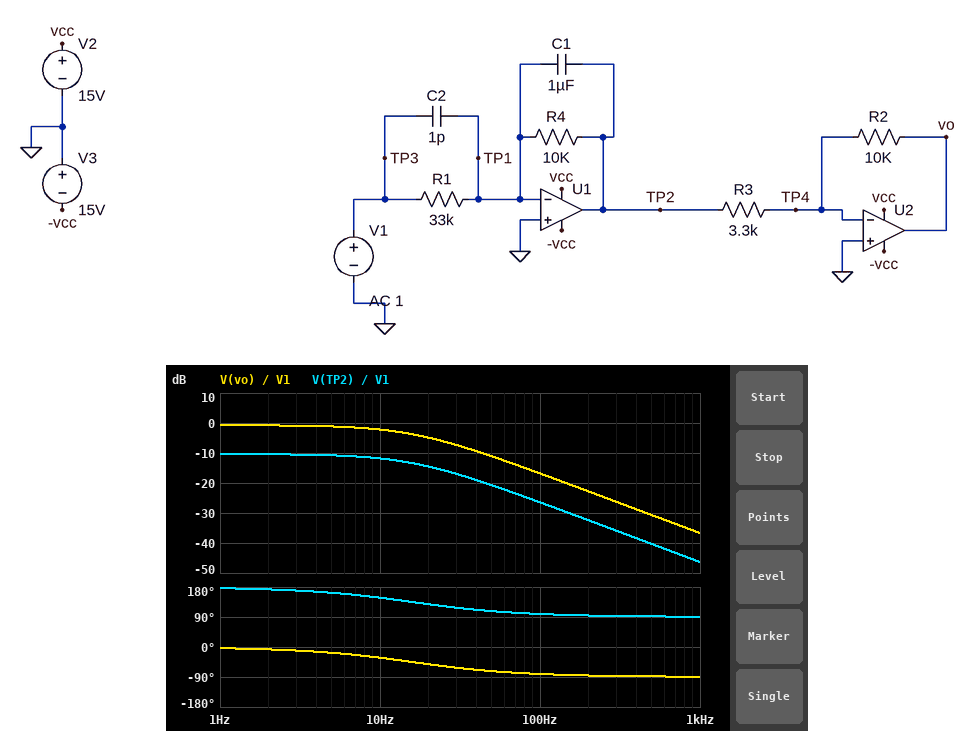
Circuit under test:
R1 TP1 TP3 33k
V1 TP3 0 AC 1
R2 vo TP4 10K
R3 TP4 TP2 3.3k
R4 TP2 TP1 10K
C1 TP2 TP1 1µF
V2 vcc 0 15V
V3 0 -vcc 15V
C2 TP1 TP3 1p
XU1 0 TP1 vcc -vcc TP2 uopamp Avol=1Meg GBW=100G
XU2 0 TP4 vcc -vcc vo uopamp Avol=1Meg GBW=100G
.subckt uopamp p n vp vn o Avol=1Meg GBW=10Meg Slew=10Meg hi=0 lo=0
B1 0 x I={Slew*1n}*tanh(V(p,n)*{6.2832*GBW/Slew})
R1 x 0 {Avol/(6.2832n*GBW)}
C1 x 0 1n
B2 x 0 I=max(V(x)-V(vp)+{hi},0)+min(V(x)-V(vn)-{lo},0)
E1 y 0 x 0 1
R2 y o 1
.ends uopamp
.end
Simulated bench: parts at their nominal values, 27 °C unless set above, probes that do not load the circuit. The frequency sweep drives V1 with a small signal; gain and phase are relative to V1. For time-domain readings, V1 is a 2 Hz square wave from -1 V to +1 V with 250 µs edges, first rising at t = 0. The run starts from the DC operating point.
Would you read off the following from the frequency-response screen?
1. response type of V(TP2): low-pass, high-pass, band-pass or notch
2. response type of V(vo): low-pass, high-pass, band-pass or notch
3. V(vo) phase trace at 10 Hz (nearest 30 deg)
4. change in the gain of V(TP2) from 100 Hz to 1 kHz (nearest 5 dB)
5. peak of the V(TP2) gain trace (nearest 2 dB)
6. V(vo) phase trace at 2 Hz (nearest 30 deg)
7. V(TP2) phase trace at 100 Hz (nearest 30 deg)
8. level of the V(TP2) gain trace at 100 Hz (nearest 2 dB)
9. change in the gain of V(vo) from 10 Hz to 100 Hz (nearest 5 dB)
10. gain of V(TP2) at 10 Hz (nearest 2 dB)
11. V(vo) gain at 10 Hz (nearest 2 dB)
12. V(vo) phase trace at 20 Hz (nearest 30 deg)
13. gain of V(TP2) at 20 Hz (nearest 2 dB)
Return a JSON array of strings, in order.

["low-pass", "low-pass", "-30 deg", "-20 dB", "-10 dB", "0 deg", "90 deg", "-26 dB", "-15 dB", "-12 dB", "-2 dB", "-60 deg", "-14 dB"]
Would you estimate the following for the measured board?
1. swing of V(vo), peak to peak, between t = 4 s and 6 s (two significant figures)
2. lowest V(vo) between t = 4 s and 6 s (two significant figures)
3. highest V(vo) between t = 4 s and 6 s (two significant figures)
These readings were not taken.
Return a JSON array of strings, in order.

["1.8 V", "-920 mV", "920 mV"]
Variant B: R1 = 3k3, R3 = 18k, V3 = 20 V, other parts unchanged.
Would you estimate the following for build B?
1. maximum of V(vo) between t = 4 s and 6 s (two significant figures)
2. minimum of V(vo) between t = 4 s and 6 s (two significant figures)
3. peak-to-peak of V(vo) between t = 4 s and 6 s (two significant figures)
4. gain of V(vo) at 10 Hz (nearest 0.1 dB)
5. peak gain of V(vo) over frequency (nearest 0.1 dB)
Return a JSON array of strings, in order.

["1.7 V", "-1.7 V", "3.4 V", "3.1 dB", "4.5 dB"]
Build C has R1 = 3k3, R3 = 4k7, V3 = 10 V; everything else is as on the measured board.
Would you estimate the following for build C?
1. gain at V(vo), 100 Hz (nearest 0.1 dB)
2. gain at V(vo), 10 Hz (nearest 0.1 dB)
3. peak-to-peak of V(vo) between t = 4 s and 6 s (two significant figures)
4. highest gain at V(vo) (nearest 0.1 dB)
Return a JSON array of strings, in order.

["0.1 dB", "14.7 dB", "13 V", "16.2 dB"]
